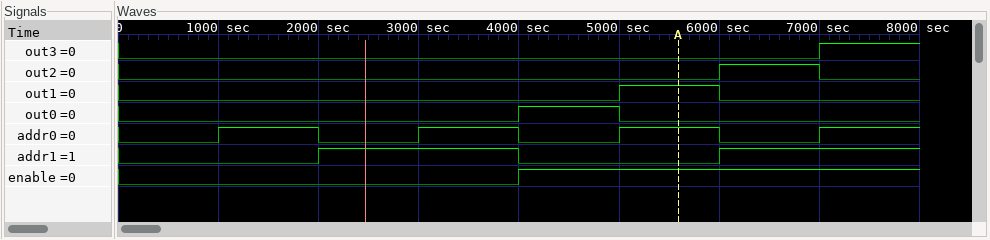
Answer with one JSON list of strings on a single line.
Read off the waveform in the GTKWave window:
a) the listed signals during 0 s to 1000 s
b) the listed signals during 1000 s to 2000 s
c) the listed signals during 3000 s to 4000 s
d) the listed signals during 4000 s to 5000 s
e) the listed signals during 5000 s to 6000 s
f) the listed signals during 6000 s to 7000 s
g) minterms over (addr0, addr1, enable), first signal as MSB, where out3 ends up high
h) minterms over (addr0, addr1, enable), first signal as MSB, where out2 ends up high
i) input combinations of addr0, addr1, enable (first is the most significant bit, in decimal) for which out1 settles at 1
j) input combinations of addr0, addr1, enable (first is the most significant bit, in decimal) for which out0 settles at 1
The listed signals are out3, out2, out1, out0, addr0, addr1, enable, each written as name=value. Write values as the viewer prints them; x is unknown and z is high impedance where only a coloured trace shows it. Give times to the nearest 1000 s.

["out3=0, out2=0, out1=0, out0=0, addr0=0, addr1=0, enable=0", "out3=0, out2=0, out1=0, out0=0, addr0=1, addr1=0, enable=0", "out3=0, out2=0, out1=0, out0=0, addr0=1, addr1=1, enable=0", "out3=0, out2=0, out1=0, out0=1, addr0=0, addr1=0, enable=1", "out3=0, out2=0, out1=1, out0=0, addr0=1, addr1=0, enable=1", "out3=0, out2=1, out1=0, out0=0, addr0=0, addr1=1, enable=1", "7", "3", "5", "1"]
